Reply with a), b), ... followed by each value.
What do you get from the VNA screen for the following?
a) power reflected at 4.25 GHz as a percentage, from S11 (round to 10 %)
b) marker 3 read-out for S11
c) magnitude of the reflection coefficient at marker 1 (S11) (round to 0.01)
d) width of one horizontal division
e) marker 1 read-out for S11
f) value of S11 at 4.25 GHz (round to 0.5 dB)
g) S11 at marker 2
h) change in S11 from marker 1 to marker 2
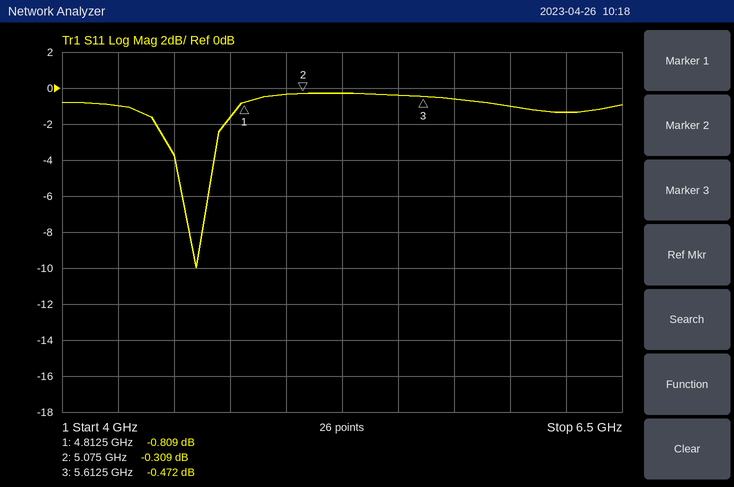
a) 80 %
b) -0.472 dB
c) 0.91
d) 250 MHz
e) -0.809 dB
f) -1.0 dB
g) -0.309 dB
h) 0.500 dB
